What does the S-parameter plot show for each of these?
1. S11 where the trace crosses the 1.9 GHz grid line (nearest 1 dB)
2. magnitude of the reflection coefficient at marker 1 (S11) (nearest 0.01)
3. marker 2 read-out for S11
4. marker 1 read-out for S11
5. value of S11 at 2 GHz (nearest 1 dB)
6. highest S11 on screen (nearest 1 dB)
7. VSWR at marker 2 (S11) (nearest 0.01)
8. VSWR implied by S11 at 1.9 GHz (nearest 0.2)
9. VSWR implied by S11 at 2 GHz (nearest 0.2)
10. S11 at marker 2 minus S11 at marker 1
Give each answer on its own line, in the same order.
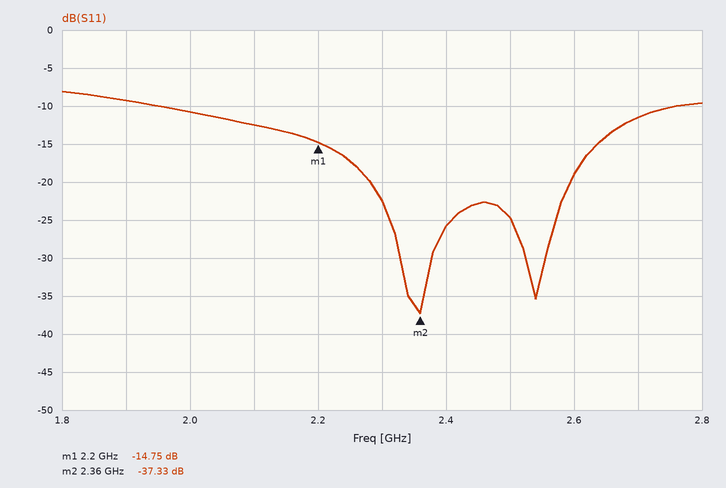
-9 dB
0.18
-37.33 dB
-14.75 dB
-11 dB
-8 dB
1.03
2.0
1.8
-22.58 dB
